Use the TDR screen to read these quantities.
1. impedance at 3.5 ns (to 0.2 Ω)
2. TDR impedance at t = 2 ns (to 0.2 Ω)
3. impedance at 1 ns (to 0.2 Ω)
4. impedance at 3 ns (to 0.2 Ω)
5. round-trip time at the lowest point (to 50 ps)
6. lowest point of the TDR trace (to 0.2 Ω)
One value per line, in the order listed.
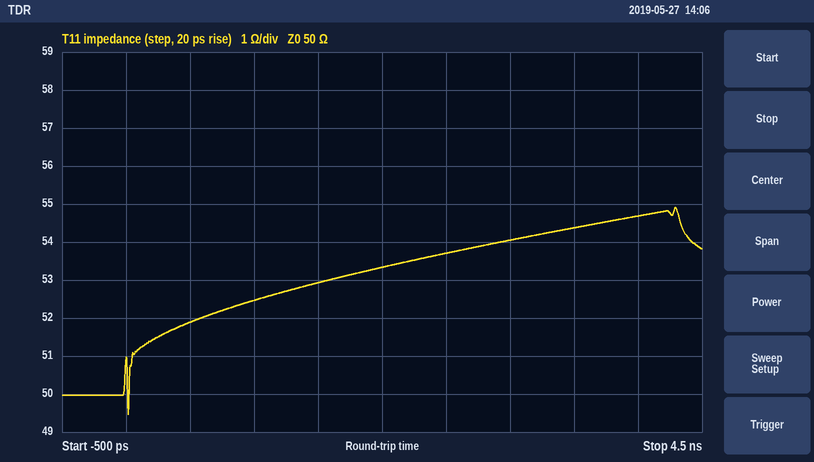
54.4 Ω
53.4 Ω
52.4 Ω
54.0 Ω
0 ps
49.4 Ω
